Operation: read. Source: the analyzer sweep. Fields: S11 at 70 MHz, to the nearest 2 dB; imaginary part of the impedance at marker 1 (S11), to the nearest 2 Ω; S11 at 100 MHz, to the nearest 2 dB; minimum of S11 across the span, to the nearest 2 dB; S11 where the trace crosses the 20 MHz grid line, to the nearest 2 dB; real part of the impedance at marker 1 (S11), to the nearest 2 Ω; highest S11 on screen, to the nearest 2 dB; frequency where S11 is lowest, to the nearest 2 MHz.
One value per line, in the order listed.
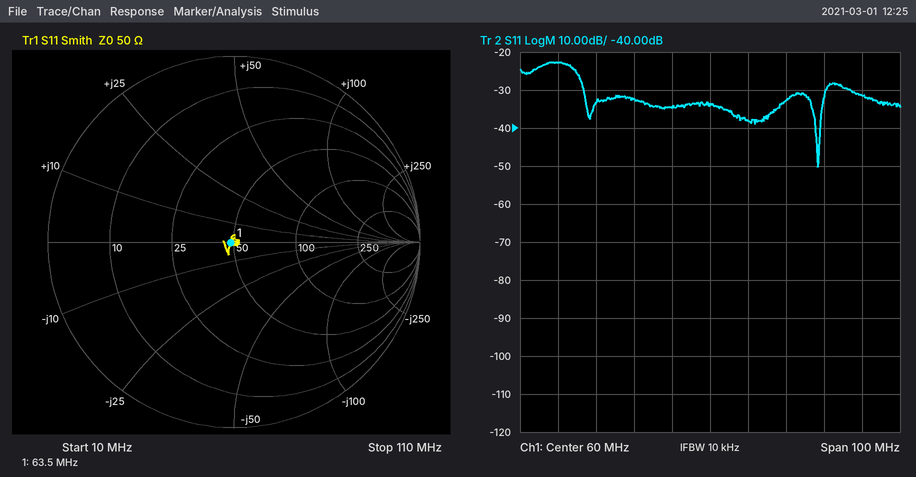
-38 dB
0 Ω
-32 dB
-50 dB
-22 dB
48 Ω
-22 dB
88 MHz
